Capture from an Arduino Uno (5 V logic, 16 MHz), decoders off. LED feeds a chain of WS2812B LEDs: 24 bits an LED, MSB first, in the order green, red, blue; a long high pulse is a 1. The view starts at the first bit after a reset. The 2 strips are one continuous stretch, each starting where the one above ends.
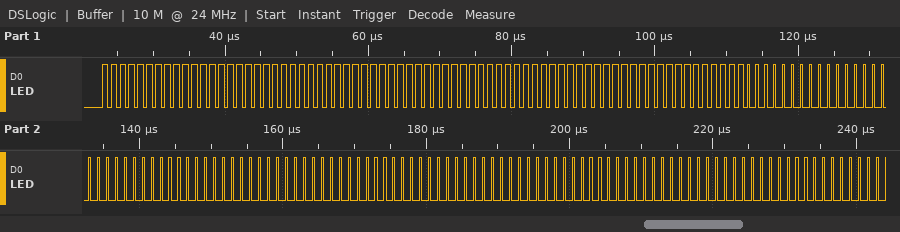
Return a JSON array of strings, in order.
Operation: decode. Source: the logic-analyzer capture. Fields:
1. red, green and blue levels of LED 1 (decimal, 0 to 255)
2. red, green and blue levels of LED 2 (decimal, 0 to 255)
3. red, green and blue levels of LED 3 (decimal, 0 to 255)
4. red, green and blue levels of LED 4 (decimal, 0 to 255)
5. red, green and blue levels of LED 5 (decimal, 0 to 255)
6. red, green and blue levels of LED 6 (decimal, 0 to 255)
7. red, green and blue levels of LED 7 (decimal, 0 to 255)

["255, 255, 255", "255, 255, 255", "255, 255, 255", "0, 0, 0", "0, 0, 0", "0, 0, 0", "0, 0, 0"]
